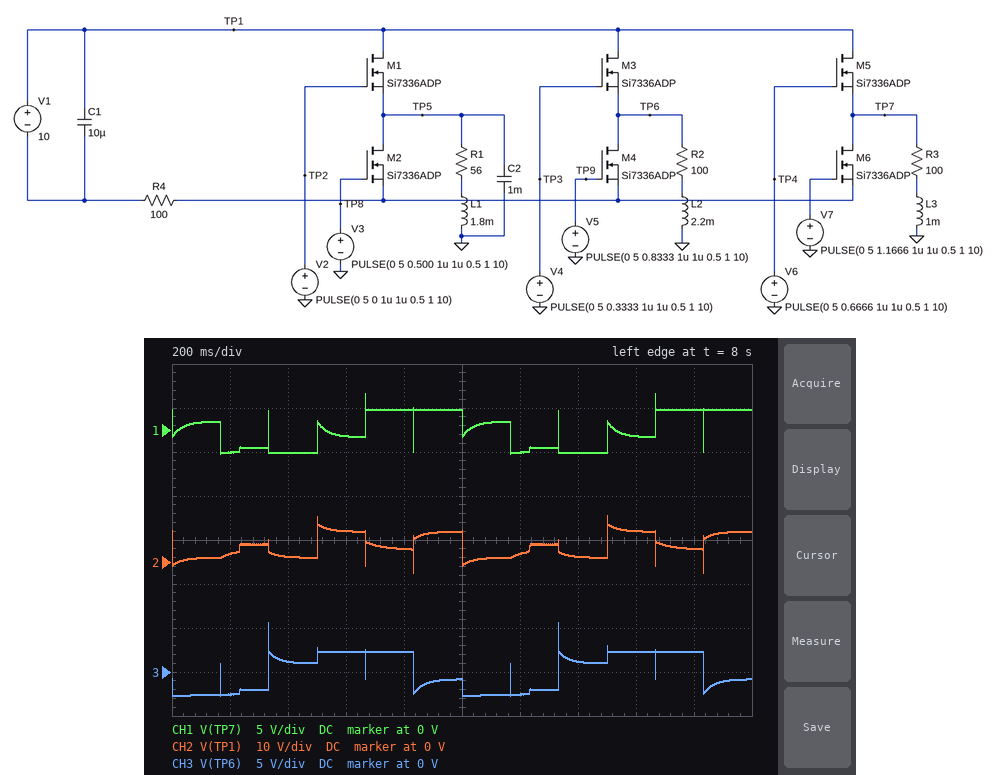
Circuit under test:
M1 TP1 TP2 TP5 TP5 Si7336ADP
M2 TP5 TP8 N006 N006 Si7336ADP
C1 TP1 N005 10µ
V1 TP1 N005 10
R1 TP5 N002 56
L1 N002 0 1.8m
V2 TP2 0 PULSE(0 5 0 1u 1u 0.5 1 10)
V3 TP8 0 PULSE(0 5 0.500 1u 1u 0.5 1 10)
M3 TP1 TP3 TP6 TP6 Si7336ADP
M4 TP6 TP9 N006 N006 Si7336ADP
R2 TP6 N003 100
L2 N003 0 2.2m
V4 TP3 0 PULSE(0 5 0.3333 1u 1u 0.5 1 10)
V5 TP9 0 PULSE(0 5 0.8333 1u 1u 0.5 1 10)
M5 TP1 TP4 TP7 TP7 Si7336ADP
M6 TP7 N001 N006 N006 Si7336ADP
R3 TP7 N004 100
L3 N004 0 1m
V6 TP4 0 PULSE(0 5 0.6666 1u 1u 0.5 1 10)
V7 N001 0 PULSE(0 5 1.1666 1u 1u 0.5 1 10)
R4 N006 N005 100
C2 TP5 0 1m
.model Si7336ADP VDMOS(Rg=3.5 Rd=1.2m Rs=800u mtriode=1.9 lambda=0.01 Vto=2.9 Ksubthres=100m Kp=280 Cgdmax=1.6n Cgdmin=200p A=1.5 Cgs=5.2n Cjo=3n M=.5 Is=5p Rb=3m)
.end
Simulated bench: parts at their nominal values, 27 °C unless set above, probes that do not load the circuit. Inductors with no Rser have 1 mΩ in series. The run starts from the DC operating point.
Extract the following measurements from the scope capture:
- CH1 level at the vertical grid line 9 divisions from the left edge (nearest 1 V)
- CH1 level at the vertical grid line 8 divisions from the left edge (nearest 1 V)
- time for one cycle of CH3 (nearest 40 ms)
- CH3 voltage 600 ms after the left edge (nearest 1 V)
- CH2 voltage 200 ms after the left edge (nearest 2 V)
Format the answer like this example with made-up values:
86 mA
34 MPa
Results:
2 V
-1 V
1.00 s
2 V
2 V
